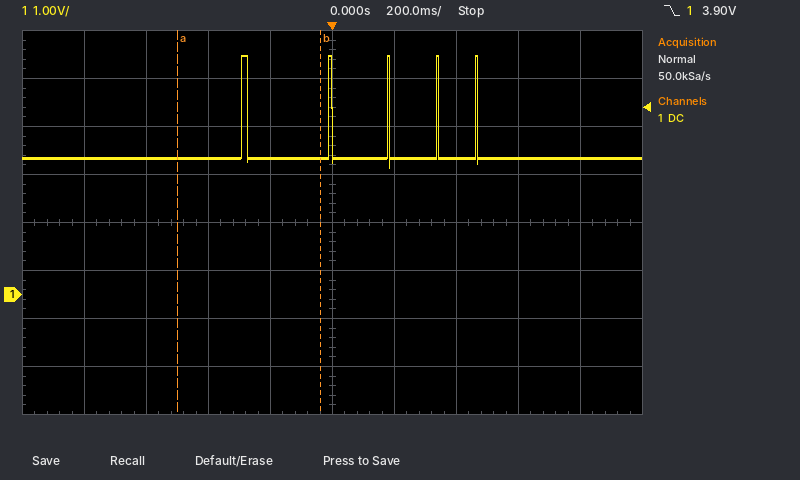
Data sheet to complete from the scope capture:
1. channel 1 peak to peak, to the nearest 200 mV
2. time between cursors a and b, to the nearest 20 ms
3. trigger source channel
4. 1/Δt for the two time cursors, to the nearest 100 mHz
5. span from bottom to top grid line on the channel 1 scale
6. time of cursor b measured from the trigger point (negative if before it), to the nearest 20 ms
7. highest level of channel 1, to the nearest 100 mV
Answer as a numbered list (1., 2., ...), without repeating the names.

1. 2.4 V
2. 460 ms
3. channel 1
4. 2.2 Hz
5. 8 V
6. -40 ms
7. 5.0 V
